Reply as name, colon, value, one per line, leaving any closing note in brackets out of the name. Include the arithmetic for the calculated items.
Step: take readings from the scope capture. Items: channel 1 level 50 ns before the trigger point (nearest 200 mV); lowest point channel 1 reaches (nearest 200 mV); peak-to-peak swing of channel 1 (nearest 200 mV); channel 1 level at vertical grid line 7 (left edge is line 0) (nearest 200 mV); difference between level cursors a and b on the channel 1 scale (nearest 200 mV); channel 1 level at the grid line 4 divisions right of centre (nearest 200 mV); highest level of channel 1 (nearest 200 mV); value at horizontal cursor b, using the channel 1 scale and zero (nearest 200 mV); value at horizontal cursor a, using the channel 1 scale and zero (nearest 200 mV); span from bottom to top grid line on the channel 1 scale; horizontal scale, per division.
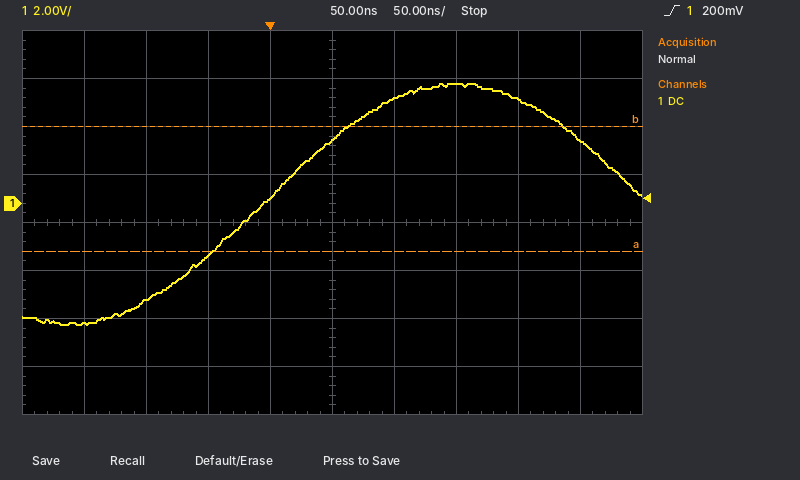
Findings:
channel 1 level 50 ns before the trigger point: -2.2 V
lowest point channel 1 reaches: -5.0 V
peak-to-peak swing of channel 1: 5.0 V − (-5.0 V) = 10.0 V
channel 1 level at vertical grid line 7 (left edge is line 0): 5.0 V
difference between level cursors a and b on the channel 1 scale: 5.2 V
channel 1 level at the grid line 4 divisions right of centre: 2.6 V
highest level of channel 1: 5.0 V
value at horizontal cursor b, using the channel 1 scale and zero: 3.2 V
value at horizontal cursor a, using the channel 1 scale and zero: -2.0 V
span from bottom to top grid line on the channel 1 scale: 16 V
horizontal scale, per division: 50 ns
